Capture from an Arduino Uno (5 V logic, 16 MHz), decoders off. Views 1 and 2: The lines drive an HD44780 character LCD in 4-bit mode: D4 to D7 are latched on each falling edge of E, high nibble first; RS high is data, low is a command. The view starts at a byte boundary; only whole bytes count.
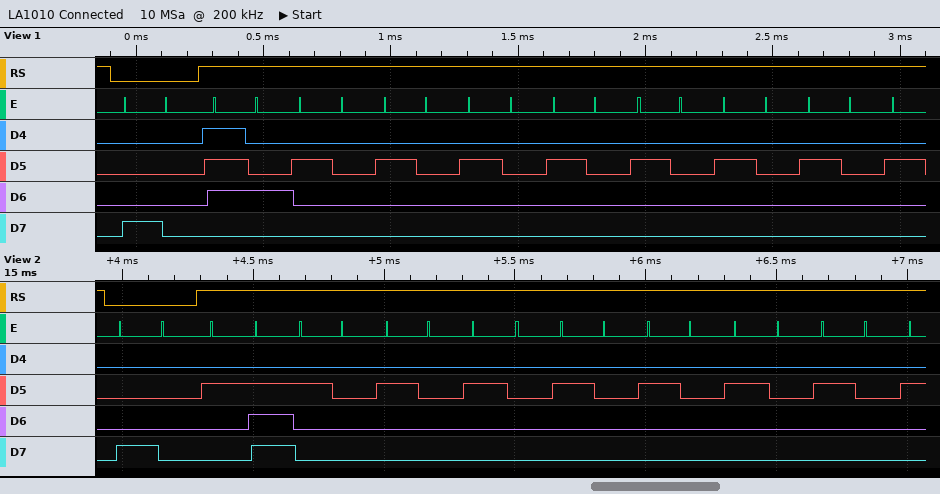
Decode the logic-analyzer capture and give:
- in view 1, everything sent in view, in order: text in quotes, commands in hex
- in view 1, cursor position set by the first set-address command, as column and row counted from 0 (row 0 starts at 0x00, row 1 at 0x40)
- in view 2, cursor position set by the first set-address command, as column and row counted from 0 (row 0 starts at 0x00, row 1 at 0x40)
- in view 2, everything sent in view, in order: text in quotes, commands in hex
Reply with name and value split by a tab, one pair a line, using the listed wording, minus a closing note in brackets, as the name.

in view 1, everything sent in view, in order: text in quotes, commands in hex	0x80 "t       "
in view 1, cursor position set by the first set-address command, as column and row counted from 0	column 0, row 0
in view 2, cursor position set by the first set-address command, as column and row counted from 0	column 0, row 0
in view 2, everything sent in view, in order: text in quotes, commands in hex	0x80 ".       "
